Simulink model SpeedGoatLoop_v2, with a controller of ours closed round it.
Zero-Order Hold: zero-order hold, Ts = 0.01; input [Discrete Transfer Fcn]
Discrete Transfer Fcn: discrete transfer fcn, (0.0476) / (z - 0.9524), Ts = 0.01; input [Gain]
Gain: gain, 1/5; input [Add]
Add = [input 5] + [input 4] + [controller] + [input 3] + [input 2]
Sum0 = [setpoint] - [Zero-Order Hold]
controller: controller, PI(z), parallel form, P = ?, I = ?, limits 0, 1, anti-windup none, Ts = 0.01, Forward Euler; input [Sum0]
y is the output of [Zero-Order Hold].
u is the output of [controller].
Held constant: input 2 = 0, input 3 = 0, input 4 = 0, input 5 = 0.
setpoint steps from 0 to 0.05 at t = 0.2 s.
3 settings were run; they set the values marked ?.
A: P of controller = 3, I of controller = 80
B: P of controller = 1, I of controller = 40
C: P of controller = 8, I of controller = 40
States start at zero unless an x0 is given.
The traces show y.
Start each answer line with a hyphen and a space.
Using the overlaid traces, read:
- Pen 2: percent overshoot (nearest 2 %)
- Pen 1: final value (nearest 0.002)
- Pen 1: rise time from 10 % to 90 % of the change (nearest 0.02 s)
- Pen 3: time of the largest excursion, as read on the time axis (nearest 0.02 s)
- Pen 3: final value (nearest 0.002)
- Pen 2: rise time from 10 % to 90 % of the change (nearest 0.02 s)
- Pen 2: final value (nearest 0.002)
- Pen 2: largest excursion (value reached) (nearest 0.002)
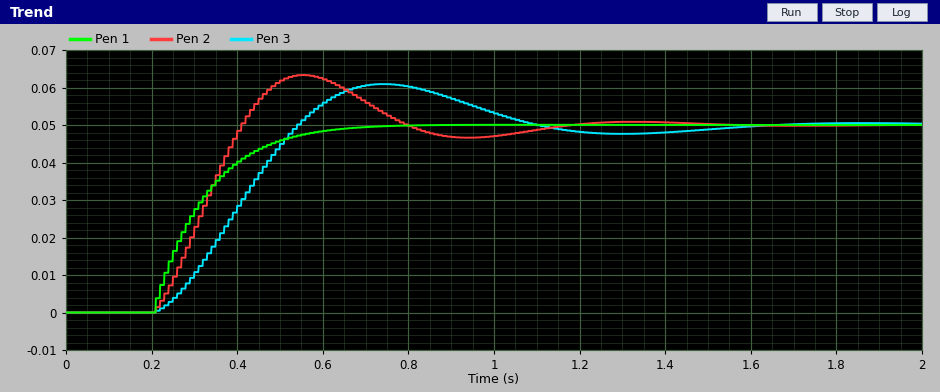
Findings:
- 26 %
- 0.050
- 0.26 s
- 0.74 s
- 0.050
- 0.16 s
- 0.050
- 0.064
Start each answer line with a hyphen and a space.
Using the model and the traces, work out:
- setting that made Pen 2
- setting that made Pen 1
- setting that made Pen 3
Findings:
- A
- C
- B
